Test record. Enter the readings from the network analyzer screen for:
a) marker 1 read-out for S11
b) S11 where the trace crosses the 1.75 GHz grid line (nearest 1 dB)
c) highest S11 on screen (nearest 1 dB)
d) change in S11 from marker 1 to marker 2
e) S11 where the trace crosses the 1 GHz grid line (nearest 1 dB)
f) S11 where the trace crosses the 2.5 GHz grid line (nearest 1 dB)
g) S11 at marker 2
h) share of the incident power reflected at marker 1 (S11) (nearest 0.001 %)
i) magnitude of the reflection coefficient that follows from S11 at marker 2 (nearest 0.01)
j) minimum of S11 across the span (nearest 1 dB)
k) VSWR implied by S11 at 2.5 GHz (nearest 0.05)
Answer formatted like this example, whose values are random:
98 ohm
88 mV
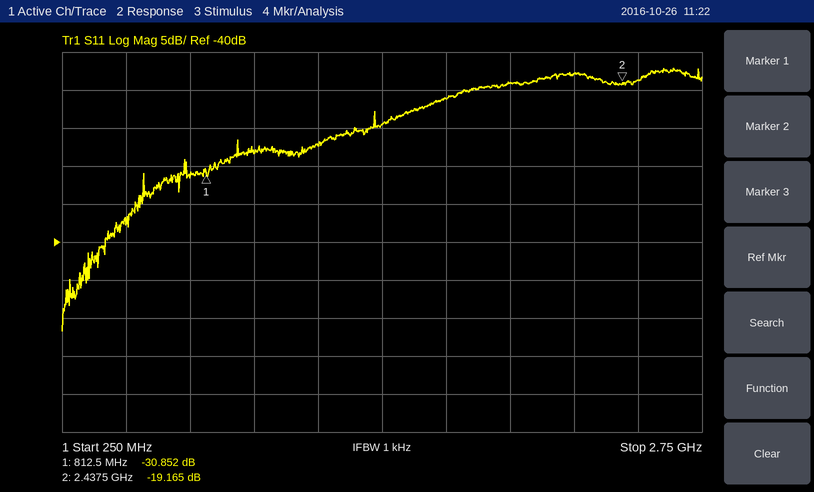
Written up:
-30.852 dB
-21 dB
-17 dB
11.687 dB
-28 dB
-19 dB
-19.165 dB
0.082 %
0.11
-52 dB
1.25
